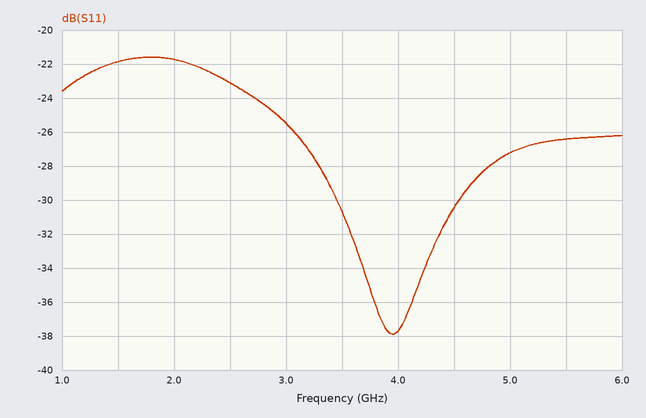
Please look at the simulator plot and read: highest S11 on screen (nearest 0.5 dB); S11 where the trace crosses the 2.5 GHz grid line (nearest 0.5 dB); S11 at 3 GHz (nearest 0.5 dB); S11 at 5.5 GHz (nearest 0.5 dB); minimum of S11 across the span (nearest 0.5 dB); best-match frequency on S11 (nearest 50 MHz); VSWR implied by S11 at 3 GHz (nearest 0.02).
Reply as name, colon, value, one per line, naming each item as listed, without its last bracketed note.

highest S11 on screen: -21.5 dB
S11 where the trace crosses the 2.5 GHz grid line: -23.0 dB
S11 at 3 GHz: -25.5 dB
S11 at 5.5 GHz: -26.5 dB
minimum of S11 across the span: -38.0 dB
best-match frequency on S11: 3.95 GHz
VSWR implied by S11 at 3 GHz: 1.12
